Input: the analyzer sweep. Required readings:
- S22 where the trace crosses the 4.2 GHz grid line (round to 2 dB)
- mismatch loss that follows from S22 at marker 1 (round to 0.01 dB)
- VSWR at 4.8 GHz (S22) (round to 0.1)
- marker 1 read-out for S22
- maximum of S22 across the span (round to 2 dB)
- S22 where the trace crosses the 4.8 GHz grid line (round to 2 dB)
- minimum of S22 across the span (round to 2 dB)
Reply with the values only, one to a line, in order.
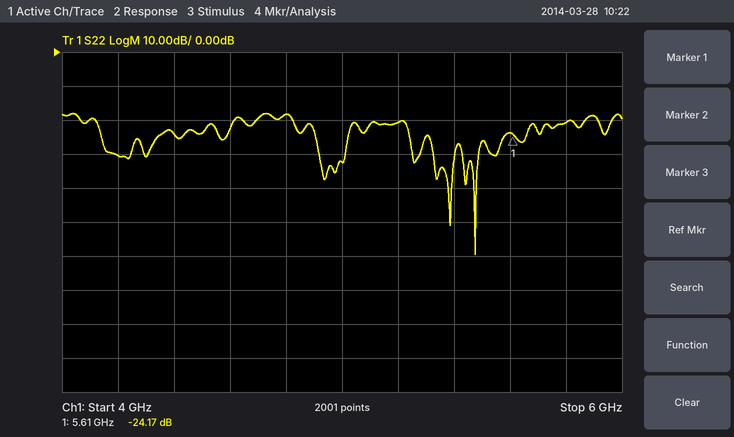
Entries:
-30 dB
0.02 dB
1.3
-24.17 dB
-18 dB
-18 dB
-60 dB
